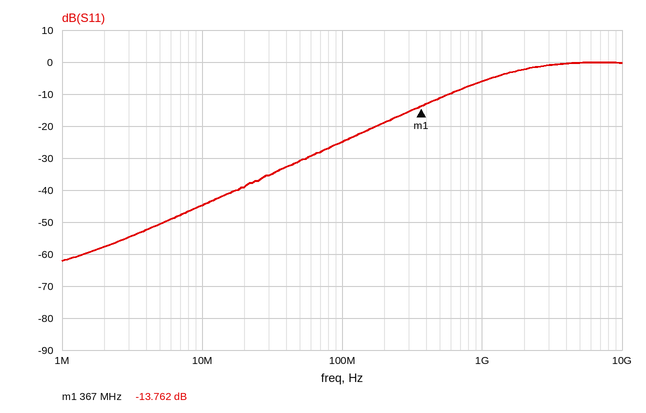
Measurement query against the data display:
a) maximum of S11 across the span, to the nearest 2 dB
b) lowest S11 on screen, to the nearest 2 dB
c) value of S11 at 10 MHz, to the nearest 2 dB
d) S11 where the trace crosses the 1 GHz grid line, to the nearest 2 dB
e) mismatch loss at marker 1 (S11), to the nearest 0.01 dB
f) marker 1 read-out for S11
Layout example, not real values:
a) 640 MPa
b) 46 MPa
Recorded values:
a) 0 dB
b) -62 dB
c) -44 dB
d) -6 dB
e) 0.19 dB
f) -13.762 dB
